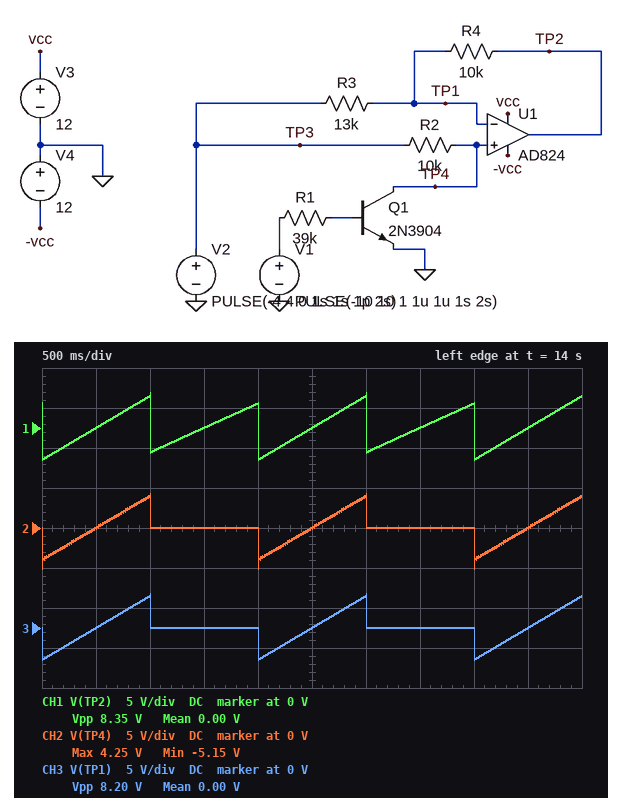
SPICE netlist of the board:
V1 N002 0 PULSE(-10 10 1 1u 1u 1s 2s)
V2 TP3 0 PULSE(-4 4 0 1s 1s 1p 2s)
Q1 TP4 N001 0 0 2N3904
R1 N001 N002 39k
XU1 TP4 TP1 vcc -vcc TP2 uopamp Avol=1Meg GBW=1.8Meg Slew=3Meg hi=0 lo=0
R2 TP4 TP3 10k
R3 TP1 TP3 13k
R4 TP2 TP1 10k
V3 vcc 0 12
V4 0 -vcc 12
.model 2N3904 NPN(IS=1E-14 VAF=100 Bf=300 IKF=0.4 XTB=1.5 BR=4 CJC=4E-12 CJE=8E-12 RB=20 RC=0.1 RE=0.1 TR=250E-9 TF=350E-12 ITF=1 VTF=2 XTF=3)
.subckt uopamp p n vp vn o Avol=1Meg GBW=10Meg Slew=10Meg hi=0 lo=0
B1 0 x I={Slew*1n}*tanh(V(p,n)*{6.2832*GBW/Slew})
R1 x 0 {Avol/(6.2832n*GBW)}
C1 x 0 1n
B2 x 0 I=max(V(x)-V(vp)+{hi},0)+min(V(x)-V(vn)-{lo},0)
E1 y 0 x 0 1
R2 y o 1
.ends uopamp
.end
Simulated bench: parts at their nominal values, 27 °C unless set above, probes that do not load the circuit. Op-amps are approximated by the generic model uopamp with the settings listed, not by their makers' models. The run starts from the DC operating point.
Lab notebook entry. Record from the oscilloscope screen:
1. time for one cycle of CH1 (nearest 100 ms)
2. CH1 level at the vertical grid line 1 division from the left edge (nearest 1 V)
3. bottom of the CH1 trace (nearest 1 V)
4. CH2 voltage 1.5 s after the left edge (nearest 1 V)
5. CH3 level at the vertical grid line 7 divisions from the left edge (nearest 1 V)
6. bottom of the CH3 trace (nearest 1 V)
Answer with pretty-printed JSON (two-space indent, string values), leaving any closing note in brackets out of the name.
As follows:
{
  "time for one cycle of CH1": "1.0 s",
  "CH1 level at the vertical grid line 1 division from the left edge": "0 V",
  "bottom of the CH1 trace": "-4 V",
  "CH2 voltage 1.5 s after the left edge": "0 V",
  "CH3 level at the vertical grid line 7 divisions from the left edge": "0 V",
  "bottom of the CH3 trace": "-4 V"
}
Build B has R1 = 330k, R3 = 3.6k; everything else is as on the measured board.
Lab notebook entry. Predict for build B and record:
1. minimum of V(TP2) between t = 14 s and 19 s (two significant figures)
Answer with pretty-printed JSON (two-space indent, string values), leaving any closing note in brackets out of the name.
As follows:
{
  "minimum of V(TP2) between t = 14 s and 19 s": "-11 V"
}
